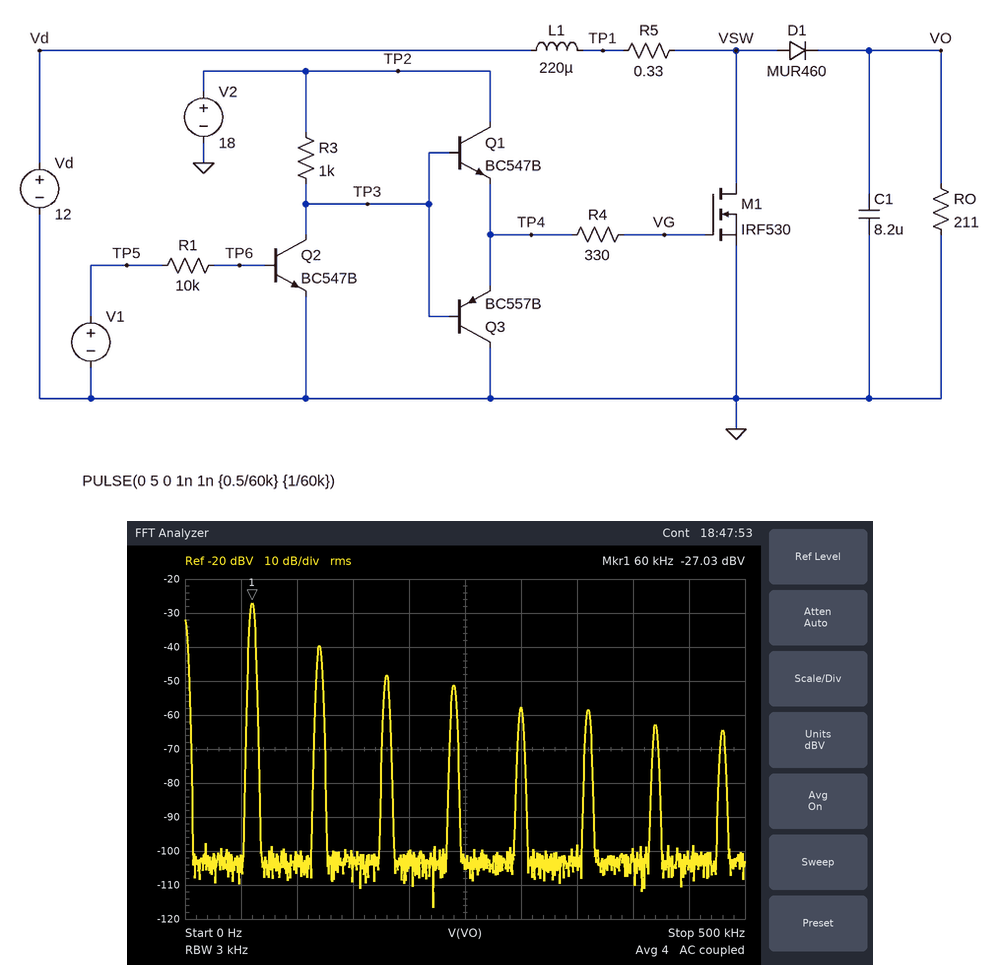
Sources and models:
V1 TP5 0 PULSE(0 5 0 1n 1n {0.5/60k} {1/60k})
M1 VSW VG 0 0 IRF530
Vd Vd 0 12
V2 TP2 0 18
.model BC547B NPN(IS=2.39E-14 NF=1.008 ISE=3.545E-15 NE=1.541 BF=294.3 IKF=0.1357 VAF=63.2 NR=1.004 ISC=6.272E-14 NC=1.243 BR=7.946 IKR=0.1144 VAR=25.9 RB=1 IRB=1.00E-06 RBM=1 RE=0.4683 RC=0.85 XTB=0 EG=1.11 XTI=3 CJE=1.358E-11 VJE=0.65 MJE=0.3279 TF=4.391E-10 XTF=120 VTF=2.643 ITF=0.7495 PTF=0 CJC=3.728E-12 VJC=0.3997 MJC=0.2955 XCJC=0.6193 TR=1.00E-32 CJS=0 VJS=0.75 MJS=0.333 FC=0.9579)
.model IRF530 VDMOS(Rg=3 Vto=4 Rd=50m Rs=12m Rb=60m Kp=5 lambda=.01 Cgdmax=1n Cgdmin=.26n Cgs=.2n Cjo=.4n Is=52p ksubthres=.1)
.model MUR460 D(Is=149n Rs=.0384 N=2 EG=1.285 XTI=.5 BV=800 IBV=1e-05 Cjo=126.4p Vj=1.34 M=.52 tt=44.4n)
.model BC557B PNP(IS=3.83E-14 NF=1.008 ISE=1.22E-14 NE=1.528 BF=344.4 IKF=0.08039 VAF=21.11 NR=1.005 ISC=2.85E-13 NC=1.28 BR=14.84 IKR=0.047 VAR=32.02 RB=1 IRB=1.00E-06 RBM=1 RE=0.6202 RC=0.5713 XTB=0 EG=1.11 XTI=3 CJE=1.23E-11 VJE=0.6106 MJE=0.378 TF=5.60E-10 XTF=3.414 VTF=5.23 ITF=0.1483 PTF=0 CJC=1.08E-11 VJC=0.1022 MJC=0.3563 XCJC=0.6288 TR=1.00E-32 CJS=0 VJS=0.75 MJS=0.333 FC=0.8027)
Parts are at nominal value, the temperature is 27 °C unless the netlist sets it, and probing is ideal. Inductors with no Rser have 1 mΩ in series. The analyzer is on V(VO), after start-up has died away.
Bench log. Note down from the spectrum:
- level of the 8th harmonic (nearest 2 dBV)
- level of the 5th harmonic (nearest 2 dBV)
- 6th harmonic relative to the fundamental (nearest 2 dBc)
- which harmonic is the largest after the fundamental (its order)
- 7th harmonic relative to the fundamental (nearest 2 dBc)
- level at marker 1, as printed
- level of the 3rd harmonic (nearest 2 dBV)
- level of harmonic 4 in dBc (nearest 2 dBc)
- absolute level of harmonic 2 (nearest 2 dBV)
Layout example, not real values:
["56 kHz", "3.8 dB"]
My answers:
["-64 dBV", "-58 dBV", "-32 dBc", "2", "-36 dBc", "-27.03 dBV", "-48 dBV", "-24 dBc", "-40 dBV"]
